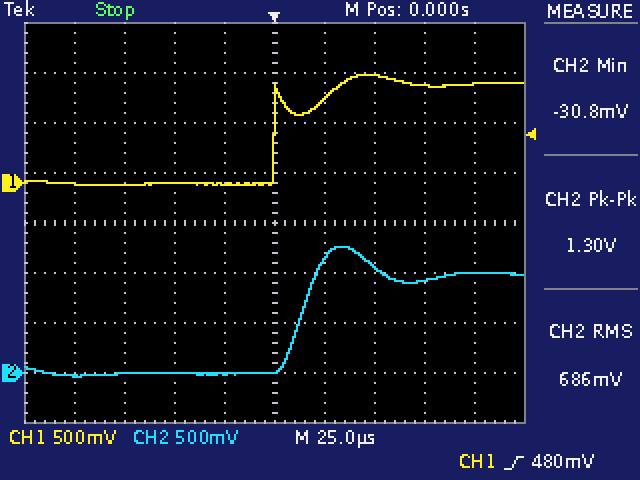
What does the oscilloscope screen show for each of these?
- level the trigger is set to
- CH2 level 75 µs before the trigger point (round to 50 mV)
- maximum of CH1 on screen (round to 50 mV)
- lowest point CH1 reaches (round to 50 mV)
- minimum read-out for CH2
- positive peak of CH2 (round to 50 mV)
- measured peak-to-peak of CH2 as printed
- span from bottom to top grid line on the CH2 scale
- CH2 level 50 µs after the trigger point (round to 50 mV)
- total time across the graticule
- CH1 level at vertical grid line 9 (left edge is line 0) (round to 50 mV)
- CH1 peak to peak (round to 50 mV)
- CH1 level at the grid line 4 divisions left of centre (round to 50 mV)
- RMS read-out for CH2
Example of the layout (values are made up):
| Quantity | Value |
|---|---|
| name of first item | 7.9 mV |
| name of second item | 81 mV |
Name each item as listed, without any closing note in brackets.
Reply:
| Quantity | Value |
|---|---|
| level the trigger is set to | 480 mV |
| CH2 level 75 µs before the trigger point | 0 mV |
| maximum of CH1 on screen | 1.10 V |
| lowest point CH1 reaches | 0 mV |
| minimum read-out for CH2 | -30.8 mV |
| positive peak of CH2 | 1.25 V |
| measured peak-to-peak of CH2 as printed | 1.30 V |
| span from bottom to top grid line on the CH2 scale | 4 V |
| CH2 level 50 µs after the trigger point | 1.05 V |
| total time across the graticule | 250 µs |
| CH1 level at vertical grid line 9 (left edge is line 0) | 1.00 V |
| CH1 peak to peak | 1.10 V |
| CH1 level at the grid line 4 divisions left of centre | 0 mV |
| RMS read-out for CH2 | 686 mV |
